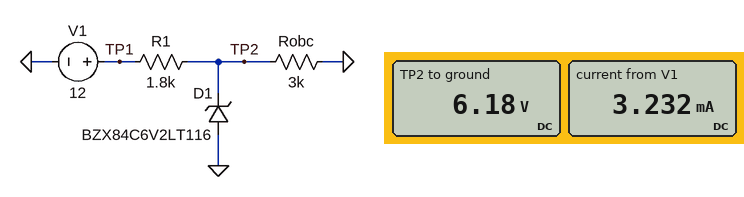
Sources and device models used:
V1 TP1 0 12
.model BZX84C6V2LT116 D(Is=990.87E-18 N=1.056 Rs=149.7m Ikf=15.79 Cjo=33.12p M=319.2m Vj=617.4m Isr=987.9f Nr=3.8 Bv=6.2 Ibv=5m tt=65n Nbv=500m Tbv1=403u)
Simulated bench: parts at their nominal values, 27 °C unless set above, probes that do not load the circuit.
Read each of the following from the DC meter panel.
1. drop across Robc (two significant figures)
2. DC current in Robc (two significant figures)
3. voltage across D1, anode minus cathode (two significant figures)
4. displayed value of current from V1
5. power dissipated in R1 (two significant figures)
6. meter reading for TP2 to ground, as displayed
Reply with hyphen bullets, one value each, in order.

- 6.2 V
- 2.1 mA
- -6.2 V
- 3.232 mA
- 19 mW
- 6.18 V
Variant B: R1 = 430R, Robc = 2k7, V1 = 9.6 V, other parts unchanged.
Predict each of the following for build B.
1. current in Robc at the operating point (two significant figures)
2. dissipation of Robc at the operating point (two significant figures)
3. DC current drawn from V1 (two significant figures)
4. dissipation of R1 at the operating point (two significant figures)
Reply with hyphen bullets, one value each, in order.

- 2.3 mA
- 14 mW
- 7.9 mA
- 27 mW
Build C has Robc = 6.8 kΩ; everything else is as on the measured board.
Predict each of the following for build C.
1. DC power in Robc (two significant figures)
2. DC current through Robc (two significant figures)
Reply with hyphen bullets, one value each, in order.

- 5.6 mW
- 910 µA
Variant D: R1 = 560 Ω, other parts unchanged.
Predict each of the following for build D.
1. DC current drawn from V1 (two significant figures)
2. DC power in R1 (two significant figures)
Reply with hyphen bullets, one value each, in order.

- 10 mA
- 60 mW
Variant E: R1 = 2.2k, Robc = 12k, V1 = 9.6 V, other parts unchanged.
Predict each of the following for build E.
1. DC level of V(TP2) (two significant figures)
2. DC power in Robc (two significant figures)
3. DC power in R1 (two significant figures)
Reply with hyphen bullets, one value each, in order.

- 6.2 V
- 3.2 mW
- 5.3 mW
